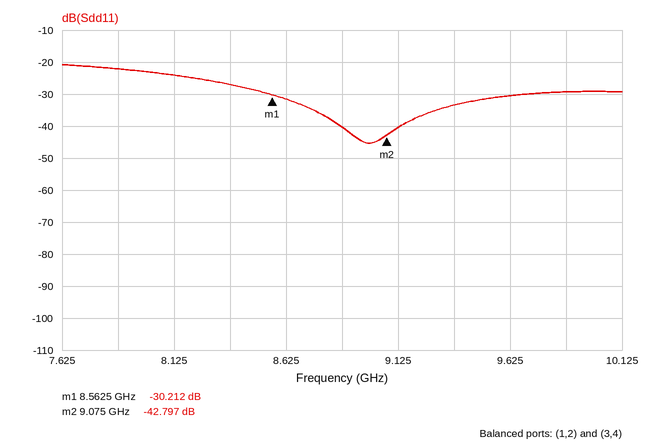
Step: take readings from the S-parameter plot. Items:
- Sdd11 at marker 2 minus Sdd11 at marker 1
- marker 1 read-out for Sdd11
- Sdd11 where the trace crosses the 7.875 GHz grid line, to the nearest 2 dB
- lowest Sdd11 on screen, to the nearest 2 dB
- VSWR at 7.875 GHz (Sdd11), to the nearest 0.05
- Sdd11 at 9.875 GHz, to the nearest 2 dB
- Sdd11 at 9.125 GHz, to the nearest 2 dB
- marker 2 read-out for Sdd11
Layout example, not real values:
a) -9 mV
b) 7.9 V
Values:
a) -12.585 dB
b) -30.212 dB
c) -22 dB
d) -46 dB
e) 1.15
f) -30 dB
g) -40 dB
h) -42.797 dB
